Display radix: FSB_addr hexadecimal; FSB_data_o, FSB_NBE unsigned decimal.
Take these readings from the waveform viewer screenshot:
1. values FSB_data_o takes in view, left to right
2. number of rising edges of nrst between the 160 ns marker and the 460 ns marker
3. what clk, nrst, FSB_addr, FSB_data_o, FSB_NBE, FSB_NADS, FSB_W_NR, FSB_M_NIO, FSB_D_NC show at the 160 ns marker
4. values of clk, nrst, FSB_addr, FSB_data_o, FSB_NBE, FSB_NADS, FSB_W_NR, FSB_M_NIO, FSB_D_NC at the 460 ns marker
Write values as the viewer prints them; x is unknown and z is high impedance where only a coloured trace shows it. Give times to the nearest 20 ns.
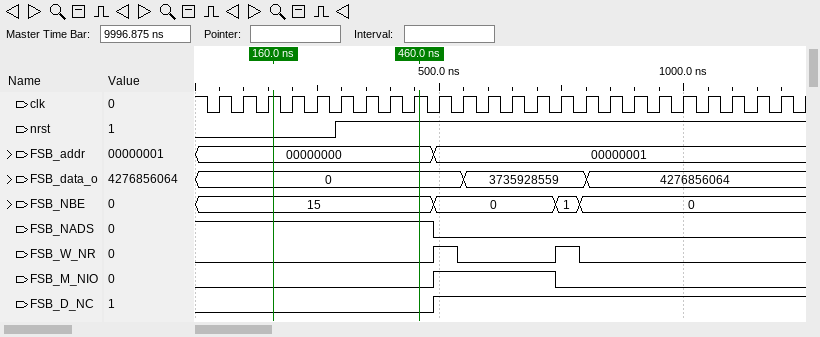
0, 3735928559, 4276856064
1
clk=1, nrst=0, FSB_addr=00000000, FSB_data_o=0, FSB_NBE=15, FSB_NADS=1, FSB_W_NR=0, FSB_M_NIO=0, FSB_D_NC=0
clk=1, nrst=1, FSB_addr=00000000, FSB_data_o=0, FSB_NBE=15, FSB_NADS=1, FSB_W_NR=0, FSB_M_NIO=0, FSB_D_NC=0
